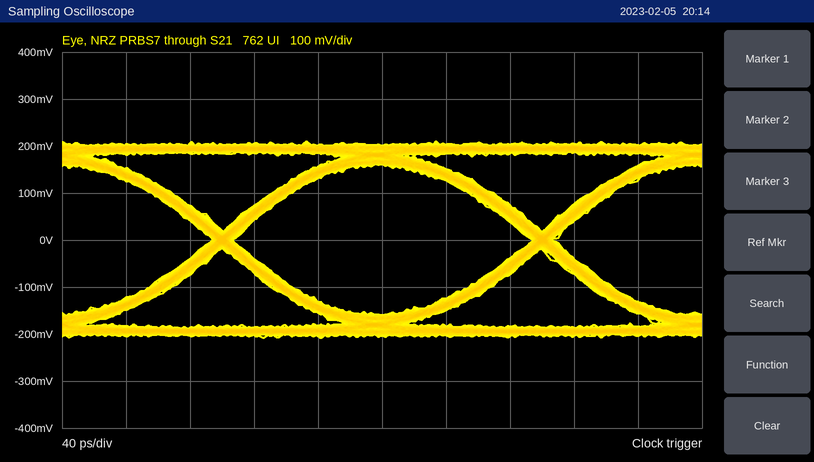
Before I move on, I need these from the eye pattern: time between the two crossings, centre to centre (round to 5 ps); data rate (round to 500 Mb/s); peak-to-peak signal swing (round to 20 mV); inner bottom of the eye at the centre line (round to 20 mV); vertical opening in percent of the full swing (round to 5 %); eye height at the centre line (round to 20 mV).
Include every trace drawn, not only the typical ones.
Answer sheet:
200 ps
5.0 Gb/s
420 mV
-160 mV
75 %
320 mV
